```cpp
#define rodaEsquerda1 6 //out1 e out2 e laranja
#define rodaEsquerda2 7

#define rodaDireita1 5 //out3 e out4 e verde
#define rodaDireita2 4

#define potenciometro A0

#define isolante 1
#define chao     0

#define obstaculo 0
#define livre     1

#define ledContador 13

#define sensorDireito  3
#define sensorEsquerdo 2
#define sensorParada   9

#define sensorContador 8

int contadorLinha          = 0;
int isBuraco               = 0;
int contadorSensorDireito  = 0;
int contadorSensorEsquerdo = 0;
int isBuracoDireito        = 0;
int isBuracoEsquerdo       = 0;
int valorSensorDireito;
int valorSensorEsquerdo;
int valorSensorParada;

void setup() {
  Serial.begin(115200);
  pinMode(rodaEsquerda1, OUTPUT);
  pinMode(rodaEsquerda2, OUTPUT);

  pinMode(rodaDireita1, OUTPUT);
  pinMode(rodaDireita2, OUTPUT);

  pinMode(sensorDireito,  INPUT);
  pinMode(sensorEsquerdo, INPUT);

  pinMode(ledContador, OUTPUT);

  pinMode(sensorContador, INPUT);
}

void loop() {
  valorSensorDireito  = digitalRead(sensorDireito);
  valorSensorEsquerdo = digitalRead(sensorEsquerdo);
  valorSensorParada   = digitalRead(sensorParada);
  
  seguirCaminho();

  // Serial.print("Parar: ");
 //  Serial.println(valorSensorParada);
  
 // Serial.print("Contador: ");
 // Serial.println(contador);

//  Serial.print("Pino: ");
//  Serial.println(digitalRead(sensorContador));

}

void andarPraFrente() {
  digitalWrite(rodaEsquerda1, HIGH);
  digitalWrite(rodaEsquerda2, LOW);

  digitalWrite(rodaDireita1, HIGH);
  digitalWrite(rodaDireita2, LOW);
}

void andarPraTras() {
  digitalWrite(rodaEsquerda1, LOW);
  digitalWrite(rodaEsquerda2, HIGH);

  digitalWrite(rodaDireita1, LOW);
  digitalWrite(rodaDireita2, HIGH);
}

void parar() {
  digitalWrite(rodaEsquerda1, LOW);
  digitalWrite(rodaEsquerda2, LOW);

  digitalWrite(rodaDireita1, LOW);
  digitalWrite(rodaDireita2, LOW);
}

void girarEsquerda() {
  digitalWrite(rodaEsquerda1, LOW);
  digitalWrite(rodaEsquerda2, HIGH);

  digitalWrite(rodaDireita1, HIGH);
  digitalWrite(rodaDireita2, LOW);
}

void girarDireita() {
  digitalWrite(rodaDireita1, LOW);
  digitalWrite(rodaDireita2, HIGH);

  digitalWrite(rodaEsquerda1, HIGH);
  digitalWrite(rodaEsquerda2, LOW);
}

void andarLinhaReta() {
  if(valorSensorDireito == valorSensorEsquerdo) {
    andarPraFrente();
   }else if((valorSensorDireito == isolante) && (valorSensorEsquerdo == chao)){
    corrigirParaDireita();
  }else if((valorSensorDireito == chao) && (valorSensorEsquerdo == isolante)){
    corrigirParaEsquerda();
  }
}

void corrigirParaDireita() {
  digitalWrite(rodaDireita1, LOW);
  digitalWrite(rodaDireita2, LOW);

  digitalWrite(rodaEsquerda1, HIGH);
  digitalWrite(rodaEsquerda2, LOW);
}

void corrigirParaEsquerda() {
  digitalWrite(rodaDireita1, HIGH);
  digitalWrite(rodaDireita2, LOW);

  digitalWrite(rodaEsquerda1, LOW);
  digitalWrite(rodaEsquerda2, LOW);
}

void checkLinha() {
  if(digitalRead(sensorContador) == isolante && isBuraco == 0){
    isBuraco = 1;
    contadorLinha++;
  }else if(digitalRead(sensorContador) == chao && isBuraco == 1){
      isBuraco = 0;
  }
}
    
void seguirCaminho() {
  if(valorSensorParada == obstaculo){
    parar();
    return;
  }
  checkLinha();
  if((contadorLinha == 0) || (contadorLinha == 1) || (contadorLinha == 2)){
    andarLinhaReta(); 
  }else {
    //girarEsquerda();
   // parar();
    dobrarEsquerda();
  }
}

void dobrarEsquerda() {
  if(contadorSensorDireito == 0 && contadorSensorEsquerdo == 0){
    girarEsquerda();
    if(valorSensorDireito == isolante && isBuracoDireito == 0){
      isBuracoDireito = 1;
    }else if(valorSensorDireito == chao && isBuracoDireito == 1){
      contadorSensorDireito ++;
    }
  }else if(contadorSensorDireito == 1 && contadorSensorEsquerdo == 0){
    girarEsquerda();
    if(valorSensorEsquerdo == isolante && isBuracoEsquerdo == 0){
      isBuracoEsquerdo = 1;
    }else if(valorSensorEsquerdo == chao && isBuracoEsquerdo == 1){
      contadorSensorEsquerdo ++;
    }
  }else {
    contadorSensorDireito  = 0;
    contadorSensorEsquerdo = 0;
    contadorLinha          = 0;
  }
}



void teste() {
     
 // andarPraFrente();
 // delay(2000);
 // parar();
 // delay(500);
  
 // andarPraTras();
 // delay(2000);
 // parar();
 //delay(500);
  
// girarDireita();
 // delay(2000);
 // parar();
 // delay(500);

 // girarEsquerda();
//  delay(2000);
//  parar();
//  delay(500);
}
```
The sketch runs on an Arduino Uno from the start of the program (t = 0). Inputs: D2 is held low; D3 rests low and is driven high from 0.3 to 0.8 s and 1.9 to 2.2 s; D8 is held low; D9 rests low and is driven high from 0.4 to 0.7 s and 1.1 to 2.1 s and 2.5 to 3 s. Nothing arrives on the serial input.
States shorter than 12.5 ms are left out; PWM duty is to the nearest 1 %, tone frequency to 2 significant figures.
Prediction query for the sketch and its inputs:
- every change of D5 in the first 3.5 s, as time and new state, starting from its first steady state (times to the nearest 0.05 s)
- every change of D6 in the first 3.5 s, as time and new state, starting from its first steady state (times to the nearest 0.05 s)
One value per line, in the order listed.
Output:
0 s low; 1.1 s high; 1.9 s low; 2.5 s high; 3 s low
0 s low; 0.4 s high; 0.7 s low; 1.1 s high; 2.1 s low; 2.5 s high; 3 s low
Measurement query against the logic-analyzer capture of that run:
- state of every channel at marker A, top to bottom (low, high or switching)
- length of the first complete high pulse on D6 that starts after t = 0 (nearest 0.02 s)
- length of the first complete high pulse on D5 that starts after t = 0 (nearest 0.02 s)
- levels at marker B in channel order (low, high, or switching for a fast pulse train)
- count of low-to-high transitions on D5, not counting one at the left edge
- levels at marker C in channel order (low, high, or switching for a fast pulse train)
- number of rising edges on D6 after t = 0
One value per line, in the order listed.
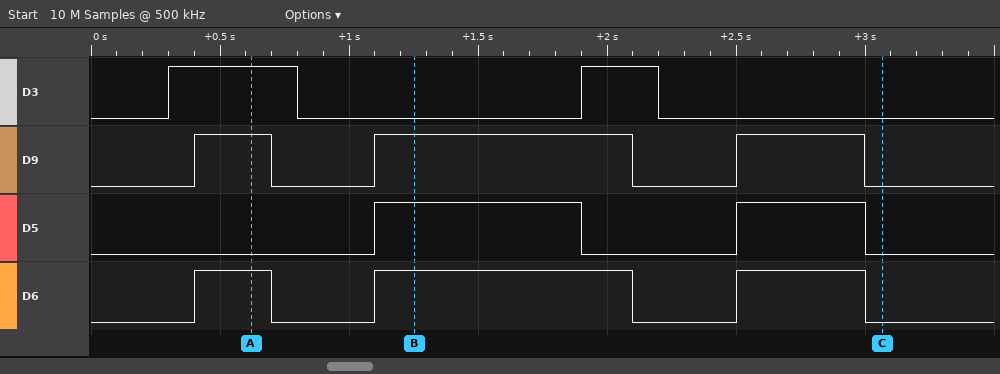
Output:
D3 high, D9 high, D5 low, D6 high
0.30 s
0.80 s
D3 low, D9 high, D5 high, D6 high
2
D3 low, D9 low, D5 low, D6 low
3
